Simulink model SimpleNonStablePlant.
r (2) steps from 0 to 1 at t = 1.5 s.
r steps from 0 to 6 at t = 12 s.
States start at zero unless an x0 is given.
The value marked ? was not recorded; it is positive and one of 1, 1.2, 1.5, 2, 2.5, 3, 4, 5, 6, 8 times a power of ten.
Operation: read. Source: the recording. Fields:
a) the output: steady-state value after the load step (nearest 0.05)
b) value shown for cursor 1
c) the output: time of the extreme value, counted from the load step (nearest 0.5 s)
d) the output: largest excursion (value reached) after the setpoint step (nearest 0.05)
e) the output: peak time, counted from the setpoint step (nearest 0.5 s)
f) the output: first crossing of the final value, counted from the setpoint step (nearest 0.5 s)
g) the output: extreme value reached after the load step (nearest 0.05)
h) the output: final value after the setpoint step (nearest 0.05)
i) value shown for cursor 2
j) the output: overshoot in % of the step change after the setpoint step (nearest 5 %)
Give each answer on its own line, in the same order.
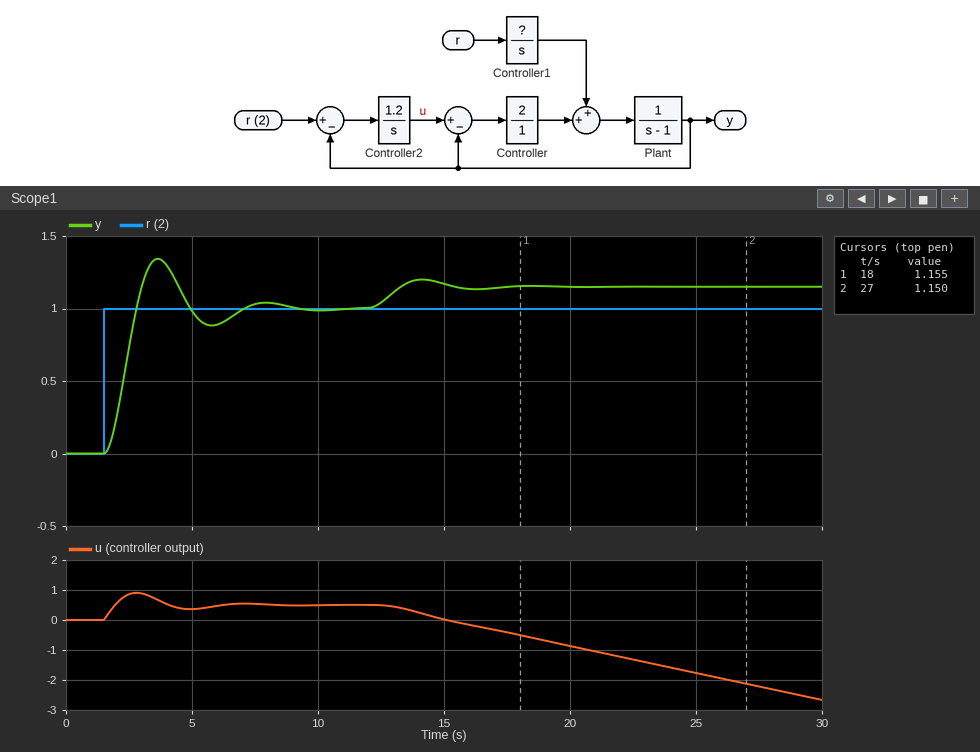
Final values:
1.15
1.155
2.0 s
1.35
2.0 s
1.5 s
1.20
1.00
1.150
35 %
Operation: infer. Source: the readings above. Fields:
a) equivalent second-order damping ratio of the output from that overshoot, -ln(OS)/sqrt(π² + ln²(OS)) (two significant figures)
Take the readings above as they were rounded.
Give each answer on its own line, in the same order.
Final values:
0.32
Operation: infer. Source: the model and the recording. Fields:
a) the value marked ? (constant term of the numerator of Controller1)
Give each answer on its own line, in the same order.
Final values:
0.06
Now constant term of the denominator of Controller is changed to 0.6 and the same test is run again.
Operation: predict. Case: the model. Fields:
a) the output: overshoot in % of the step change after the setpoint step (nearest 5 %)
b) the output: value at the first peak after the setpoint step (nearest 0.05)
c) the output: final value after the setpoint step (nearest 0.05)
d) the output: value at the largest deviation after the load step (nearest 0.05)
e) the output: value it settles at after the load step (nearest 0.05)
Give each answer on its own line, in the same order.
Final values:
10 %
1.10
1.00
1.10
1.10
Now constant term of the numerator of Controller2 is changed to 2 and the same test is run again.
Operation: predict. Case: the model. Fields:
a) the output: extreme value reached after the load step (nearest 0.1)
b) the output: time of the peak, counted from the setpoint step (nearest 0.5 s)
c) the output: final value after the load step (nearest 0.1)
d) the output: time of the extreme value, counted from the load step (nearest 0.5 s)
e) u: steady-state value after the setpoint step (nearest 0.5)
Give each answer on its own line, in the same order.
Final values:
1.1
1.5 s
1.1
1.5 s
0.5
